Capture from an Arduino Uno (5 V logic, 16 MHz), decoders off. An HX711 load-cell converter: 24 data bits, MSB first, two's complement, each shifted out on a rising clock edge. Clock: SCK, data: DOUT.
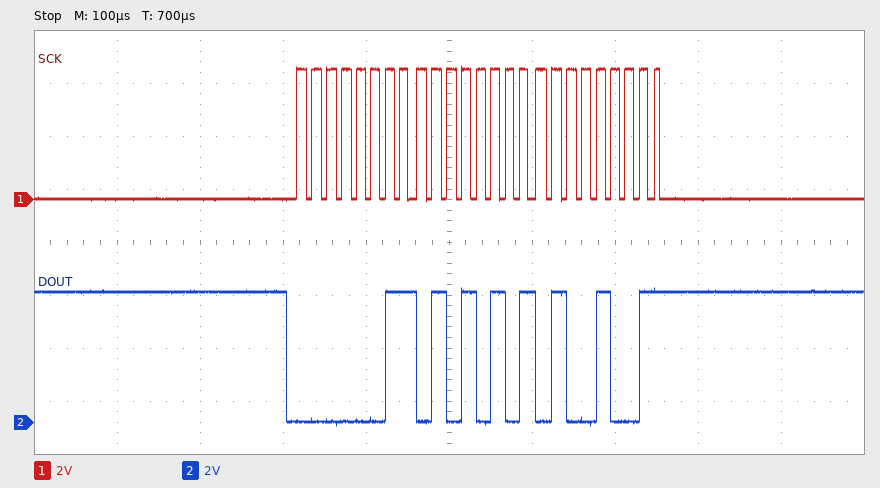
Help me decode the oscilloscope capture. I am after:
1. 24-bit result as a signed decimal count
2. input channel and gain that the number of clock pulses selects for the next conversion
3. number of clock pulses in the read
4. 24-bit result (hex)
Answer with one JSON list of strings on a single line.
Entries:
["218441", "channel A, gain 128", "25", "0x035549"]
